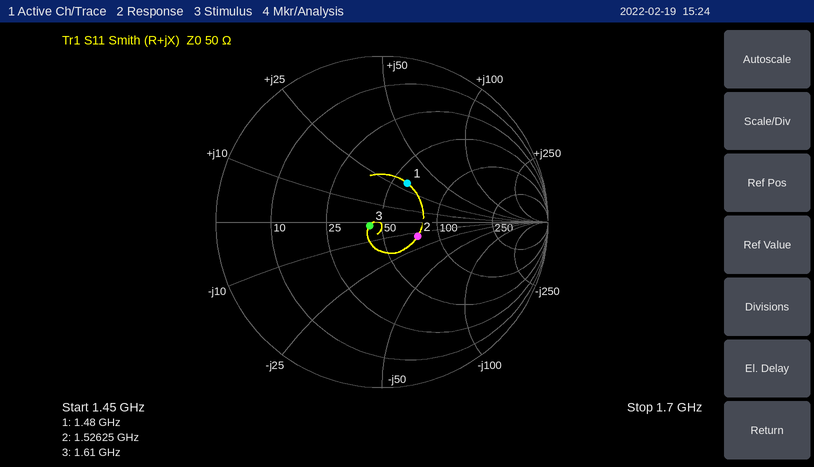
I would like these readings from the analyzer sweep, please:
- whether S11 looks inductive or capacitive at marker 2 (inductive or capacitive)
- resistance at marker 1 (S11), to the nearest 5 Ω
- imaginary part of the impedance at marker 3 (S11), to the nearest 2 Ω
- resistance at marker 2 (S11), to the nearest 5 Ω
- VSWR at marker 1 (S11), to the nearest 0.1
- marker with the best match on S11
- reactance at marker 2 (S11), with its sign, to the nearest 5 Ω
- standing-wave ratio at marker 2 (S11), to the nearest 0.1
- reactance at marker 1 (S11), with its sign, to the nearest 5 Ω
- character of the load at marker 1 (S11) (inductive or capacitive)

capacitive
60 Ω
-2 Ω
75 Ω
1.8
marker 3
-15 Ω
1.6
+30 Ω
inductive
